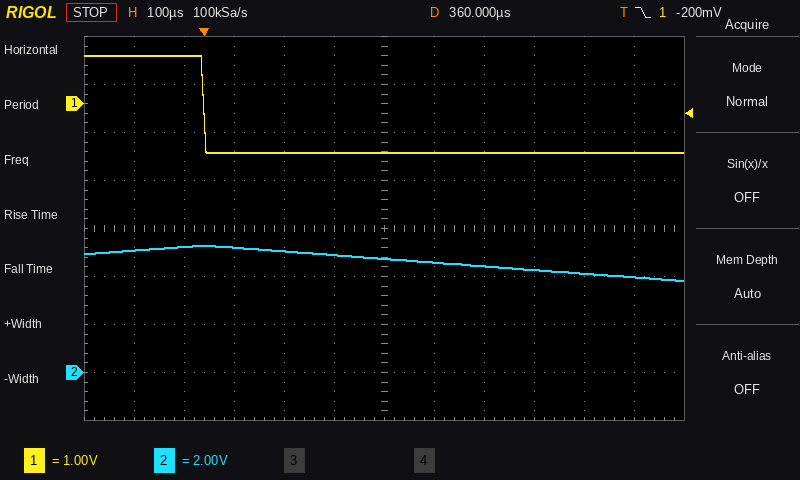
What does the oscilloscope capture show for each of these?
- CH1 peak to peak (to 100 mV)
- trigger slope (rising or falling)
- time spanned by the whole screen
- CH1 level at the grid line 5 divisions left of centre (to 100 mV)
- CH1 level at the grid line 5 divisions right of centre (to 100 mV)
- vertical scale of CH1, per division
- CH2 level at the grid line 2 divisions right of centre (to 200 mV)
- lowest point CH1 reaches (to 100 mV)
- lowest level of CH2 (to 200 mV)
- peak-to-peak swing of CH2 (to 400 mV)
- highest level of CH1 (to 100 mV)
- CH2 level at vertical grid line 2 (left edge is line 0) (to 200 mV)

2.0 V
falling
1.2 ms
1.0 V
-1.0 V
1 V
4.4 V
-1.0 V
3.8 V
1.6 V
1.0 V
5.2 V
